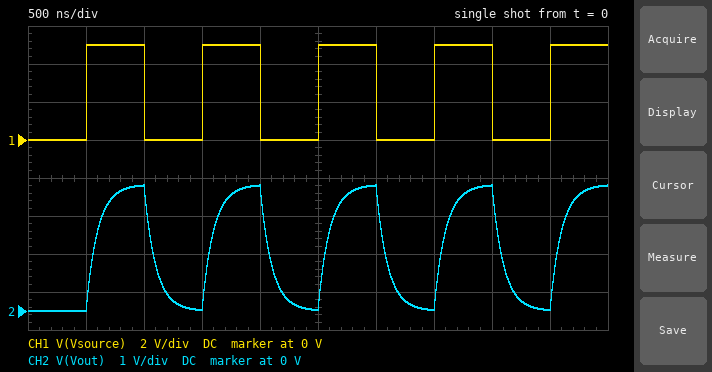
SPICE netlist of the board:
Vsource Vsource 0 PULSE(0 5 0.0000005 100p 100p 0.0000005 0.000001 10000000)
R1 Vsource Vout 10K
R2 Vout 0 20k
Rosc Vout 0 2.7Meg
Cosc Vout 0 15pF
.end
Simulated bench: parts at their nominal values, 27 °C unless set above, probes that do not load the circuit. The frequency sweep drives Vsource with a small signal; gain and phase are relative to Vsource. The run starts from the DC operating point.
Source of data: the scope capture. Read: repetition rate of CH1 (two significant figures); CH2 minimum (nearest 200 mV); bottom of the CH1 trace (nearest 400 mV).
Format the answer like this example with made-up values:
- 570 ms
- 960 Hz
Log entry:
- 1.0 MHz
- 0 V
- 0 V
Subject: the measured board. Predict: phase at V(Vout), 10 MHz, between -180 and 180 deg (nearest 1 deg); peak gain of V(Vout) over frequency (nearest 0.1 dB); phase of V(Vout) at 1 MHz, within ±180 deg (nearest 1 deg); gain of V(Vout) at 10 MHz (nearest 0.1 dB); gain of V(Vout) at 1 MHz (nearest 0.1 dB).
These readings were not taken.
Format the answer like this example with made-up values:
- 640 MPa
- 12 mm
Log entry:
- -81 deg
- -3.5 dB
- -32 deg
- -19.6 dB
- -5.0 dB
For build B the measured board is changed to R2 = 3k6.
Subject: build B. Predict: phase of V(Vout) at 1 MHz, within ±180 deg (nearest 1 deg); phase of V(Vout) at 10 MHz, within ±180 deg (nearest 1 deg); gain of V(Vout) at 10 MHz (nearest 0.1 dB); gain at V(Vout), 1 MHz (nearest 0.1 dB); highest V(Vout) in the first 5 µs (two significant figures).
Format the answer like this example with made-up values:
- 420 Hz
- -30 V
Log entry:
- -14 deg
- -68 deg
- -20.1 dB
- -11.8 dB
- 1.3 V
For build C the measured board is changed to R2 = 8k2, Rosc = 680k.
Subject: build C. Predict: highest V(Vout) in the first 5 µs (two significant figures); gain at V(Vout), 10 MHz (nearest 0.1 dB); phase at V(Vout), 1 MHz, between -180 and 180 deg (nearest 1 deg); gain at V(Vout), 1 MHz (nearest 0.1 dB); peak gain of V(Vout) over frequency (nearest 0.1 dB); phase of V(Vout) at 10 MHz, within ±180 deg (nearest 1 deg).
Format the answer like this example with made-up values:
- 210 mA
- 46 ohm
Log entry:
- 2.2 V
- -19.7 dB
- -23 deg
- -7.7 dB
- -7.0 dB
- -77 deg
